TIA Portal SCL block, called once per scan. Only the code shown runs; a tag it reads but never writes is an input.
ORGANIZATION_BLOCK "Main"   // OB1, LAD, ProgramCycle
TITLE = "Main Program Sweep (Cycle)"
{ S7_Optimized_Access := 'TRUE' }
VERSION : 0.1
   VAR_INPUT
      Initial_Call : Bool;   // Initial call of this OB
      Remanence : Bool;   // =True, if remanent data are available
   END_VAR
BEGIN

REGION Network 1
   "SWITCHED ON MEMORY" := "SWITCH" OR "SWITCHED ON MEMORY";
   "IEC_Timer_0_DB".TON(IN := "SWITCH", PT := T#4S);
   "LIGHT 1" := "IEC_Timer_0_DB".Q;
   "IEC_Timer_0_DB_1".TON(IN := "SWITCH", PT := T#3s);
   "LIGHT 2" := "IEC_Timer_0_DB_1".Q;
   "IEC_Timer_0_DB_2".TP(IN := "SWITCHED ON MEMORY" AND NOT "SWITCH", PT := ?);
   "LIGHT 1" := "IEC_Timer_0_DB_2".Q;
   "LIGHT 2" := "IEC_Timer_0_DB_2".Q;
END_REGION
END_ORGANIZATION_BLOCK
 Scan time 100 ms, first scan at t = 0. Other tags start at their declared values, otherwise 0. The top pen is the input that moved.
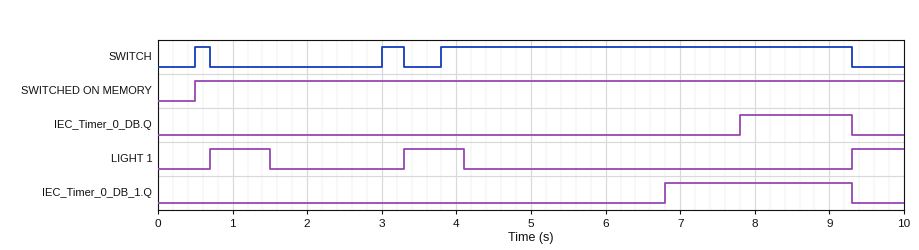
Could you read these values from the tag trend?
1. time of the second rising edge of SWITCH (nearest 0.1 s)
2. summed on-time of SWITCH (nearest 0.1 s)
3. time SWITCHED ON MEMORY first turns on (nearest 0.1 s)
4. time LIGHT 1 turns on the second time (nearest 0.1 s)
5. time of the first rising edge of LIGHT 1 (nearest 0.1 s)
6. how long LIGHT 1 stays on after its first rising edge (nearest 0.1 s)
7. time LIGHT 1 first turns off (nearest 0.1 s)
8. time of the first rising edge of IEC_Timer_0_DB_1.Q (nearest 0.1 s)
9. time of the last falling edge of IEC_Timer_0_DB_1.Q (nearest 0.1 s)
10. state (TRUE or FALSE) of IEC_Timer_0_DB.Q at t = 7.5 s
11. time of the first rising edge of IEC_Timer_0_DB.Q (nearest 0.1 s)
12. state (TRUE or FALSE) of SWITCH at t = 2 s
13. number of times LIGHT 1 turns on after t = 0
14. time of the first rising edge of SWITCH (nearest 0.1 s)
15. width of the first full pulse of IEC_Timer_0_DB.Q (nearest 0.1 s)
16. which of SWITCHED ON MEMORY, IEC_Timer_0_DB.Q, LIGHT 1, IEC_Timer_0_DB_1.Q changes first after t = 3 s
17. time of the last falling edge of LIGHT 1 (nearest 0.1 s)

3.0 s
6.0 s
0.5 s
3.3 s
0.7 s
0.8 s
1.5 s
6.8 s
9.3 s
FALSE
7.8 s
FALSE
3
0.5 s
1.5 s
LIGHT 1
4.1 s
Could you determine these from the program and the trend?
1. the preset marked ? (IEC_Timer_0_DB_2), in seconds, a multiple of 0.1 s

0.8 s
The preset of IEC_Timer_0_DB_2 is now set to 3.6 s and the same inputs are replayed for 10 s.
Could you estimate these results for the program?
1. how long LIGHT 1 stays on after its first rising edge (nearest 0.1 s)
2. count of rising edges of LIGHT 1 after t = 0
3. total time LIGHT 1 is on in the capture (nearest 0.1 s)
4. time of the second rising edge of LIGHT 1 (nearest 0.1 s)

3.6 s
2
4.3 s
9.3 s
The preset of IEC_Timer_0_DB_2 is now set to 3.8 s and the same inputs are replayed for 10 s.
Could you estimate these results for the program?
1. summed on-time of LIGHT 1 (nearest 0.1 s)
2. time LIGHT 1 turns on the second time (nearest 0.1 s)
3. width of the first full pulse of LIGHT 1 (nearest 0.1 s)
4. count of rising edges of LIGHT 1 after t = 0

4.5 s
9.3 s
3.8 s
2
